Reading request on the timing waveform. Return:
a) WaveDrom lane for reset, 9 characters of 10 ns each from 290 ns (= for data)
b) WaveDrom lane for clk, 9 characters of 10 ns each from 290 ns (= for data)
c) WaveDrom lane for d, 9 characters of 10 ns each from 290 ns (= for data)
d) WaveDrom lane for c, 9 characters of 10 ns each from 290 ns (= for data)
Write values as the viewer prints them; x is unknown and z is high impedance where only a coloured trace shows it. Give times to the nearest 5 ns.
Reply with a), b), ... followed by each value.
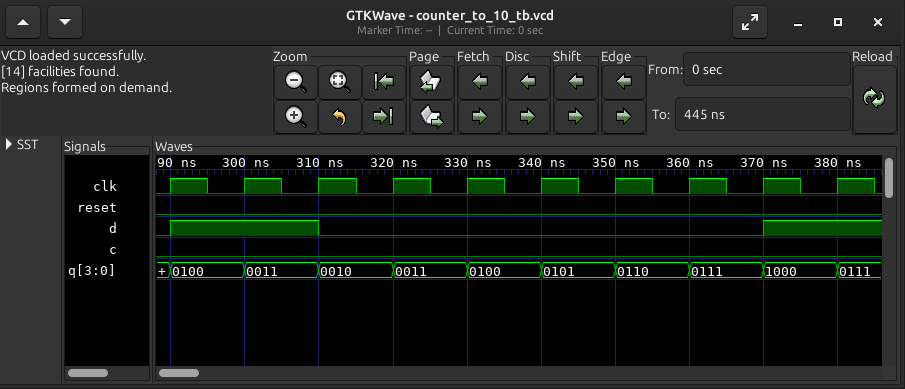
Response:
a) {name: 'reset', wave: '0........'}
b) {name: 'clk', wave: 'p........'}
c) {name: 'd', wave: '1.0.....1'}
d) {name: 'c', wave: '0........'}
